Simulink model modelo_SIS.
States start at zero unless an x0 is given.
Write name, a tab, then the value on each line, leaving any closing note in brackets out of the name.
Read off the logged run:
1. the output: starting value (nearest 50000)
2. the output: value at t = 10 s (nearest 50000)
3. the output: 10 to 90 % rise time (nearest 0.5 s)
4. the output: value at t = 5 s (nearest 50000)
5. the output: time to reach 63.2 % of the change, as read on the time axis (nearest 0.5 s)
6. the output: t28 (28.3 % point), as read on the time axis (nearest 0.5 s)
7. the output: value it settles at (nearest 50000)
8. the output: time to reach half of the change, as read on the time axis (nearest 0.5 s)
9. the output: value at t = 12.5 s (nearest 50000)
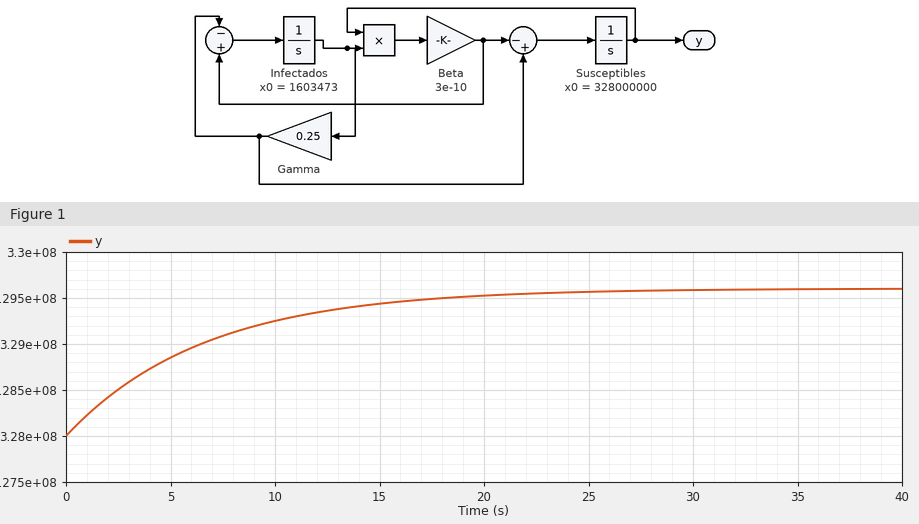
the output: starting value	328000000
the output: value at t = 10 s	329250000
the output: 10 to 90 % rise time	14.5 s
the output: value at t = 5 s	328850000
the output: time to reach 63.2 % of the change, as read on the time axis	6.5 s
the output: t28 (28.3 % point), as read on the time axis	2.0 s
the output: value it settles at	329600000
the output: time to reach half of the change, as read on the time axis	4.5 s
the output: value at t = 12.5 s	329350000
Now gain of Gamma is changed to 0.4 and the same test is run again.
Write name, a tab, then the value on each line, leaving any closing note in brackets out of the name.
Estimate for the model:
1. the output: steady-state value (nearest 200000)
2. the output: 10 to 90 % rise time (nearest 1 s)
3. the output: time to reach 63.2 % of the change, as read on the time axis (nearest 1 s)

the output: steady-state value	329600000
the output: 10 to 90 % rise time	7 s
the output: time to reach 63.2 % of the change, as read on the time axis	3 s
